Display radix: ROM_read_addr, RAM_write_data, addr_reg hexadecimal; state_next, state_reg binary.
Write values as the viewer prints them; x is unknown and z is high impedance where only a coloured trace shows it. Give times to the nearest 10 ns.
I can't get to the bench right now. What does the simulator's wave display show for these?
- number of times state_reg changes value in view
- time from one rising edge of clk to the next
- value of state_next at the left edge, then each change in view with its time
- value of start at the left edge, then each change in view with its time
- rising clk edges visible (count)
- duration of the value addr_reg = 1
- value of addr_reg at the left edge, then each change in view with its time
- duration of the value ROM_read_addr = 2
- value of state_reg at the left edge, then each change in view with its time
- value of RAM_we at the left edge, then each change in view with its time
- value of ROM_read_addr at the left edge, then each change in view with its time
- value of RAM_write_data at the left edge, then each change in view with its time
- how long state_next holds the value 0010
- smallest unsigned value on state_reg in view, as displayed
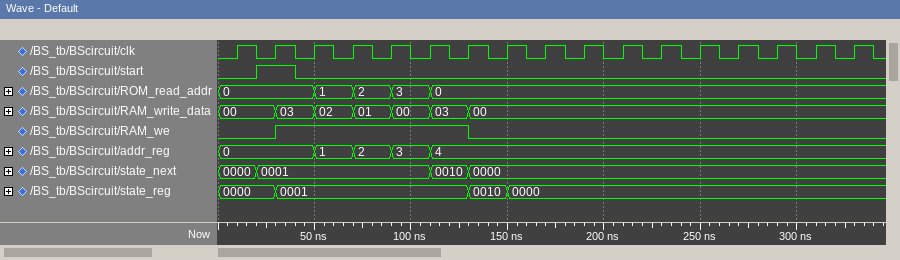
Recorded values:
3
20 ns
0000, 0001 at 20 ns, 0010 at 110 ns, 0000 at 130 ns
0, 1 at 20 ns, 0 at 40 ns
17
20 ns
0, 1 at 50 ns, 2 at 70 ns, 3 at 90 ns, 4 at 110 ns
20 ns
0000, 0001 at 30 ns, 0010 at 130 ns, 0000 at 150 ns
0, 1 at 30 ns, 0 at 130 ns
0, 1 at 50 ns, 2 at 70 ns, 3 at 90 ns, 0 at 110 ns
00, 03 at 30 ns, 02 at 50 ns, 01 at 70 ns, 00 at 90 ns, 03 at 110 ns, 00 at 130 ns
20 ns
0000
